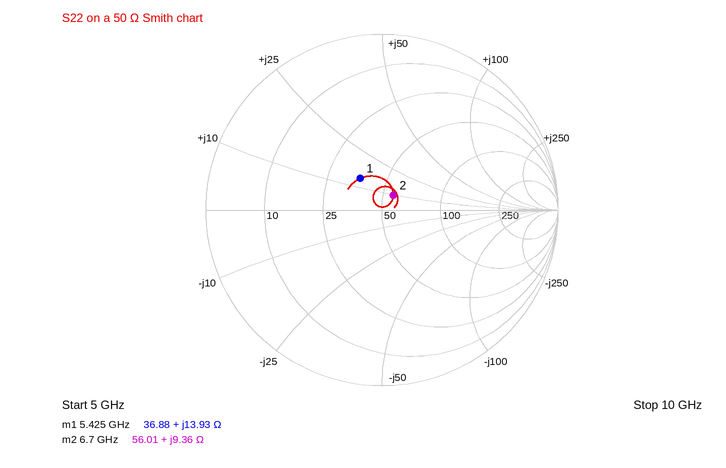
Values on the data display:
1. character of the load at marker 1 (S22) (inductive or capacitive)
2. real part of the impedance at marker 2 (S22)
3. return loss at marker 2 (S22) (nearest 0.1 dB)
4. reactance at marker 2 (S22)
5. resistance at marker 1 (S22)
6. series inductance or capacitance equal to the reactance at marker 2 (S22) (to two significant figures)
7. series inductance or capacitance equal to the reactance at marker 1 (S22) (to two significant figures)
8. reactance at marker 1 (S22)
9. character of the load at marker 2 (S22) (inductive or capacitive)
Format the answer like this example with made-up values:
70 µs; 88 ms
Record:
inductive; 56.01 Ω; 19.6 dB; +9.36 Ω; 36.88 Ω; 220 pH; 410 pH; +13.93 Ω; inductive
